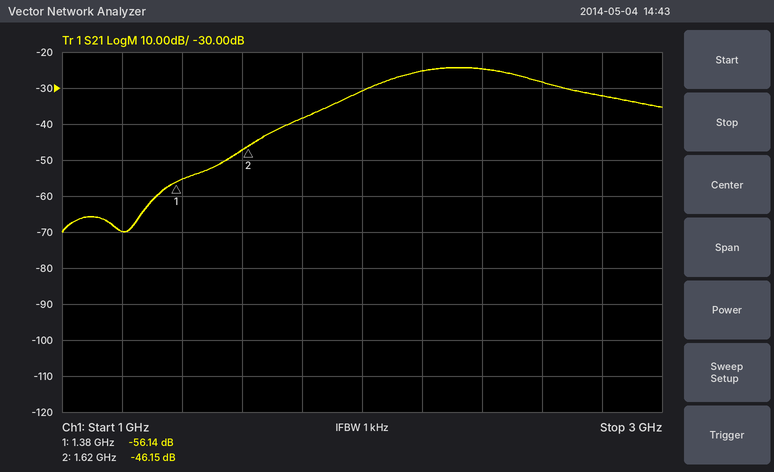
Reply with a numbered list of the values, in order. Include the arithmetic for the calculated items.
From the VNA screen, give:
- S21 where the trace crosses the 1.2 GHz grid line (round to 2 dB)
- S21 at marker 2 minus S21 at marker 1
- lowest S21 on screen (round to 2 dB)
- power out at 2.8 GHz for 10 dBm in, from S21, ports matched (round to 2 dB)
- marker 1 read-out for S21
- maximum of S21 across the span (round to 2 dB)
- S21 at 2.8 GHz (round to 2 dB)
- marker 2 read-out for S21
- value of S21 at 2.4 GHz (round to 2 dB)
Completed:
1. -70 dB
2. -46.15 − (-56.14) = 9.99 dB
3. -70 dB
4. 10 dBm + (-32 dB) = -22 dBm
5. -56.14 dB
6. -24 dB
7. -32 dB
8. -46.15 dB
9. -24 dB
